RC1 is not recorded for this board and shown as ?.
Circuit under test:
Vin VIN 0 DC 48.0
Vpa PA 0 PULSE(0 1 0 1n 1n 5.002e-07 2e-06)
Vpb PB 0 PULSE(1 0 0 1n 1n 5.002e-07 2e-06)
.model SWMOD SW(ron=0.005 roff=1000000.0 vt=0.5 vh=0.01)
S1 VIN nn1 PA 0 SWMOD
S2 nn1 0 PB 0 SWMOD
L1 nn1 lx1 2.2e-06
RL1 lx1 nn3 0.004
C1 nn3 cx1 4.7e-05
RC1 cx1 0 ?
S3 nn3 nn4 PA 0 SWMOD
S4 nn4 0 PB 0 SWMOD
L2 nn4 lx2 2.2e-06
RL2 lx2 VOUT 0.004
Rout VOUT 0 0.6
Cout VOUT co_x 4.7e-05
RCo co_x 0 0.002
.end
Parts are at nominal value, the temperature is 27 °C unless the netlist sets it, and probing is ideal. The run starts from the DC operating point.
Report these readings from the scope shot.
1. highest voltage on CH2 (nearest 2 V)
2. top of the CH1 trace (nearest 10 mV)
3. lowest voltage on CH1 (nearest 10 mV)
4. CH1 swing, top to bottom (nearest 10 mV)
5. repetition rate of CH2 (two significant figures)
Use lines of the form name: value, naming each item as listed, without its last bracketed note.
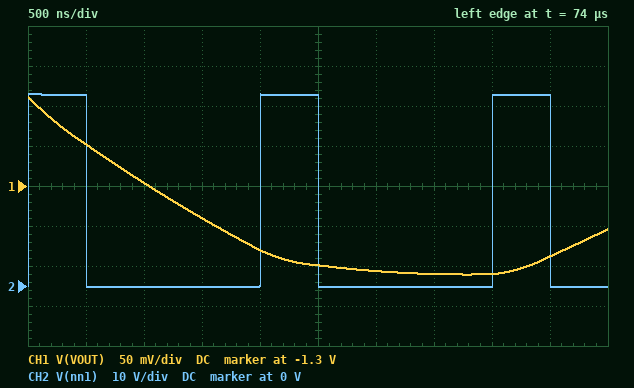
highest voltage on CH2: 48 V
top of the CH1 trace: -1.19 V
lowest voltage on CH1: -1.41 V
CH1 swing, top to bottom: 220 mV
repetition rate of CH2: 500 kHz
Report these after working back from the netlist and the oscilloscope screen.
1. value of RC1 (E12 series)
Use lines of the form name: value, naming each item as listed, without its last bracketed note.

value of RC1: 4.7 mΩ
